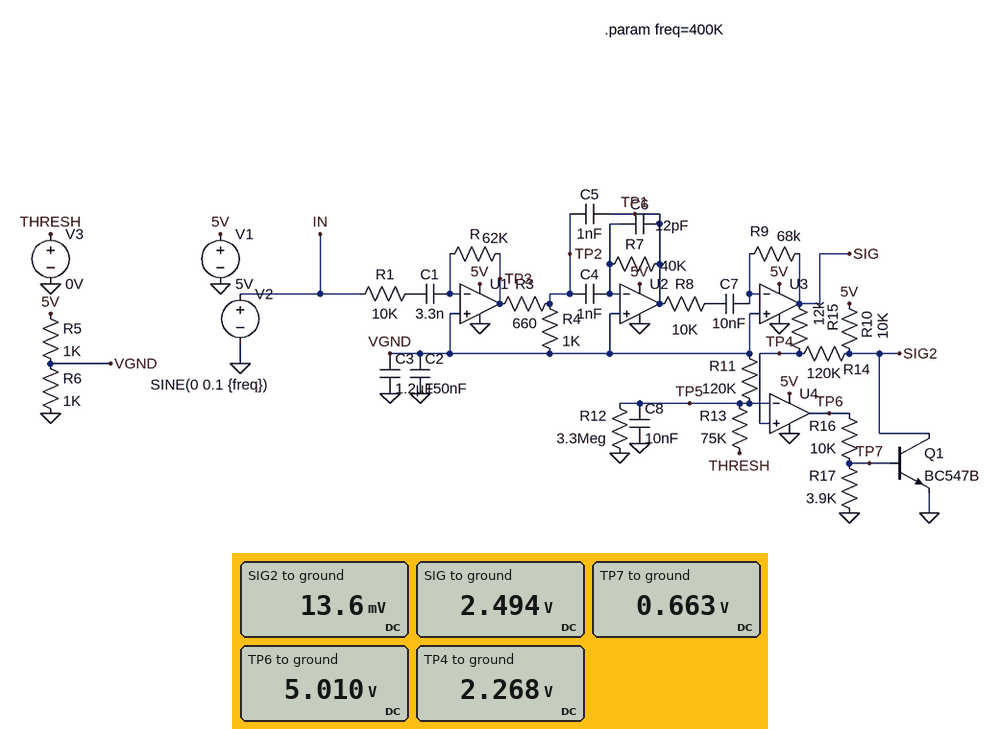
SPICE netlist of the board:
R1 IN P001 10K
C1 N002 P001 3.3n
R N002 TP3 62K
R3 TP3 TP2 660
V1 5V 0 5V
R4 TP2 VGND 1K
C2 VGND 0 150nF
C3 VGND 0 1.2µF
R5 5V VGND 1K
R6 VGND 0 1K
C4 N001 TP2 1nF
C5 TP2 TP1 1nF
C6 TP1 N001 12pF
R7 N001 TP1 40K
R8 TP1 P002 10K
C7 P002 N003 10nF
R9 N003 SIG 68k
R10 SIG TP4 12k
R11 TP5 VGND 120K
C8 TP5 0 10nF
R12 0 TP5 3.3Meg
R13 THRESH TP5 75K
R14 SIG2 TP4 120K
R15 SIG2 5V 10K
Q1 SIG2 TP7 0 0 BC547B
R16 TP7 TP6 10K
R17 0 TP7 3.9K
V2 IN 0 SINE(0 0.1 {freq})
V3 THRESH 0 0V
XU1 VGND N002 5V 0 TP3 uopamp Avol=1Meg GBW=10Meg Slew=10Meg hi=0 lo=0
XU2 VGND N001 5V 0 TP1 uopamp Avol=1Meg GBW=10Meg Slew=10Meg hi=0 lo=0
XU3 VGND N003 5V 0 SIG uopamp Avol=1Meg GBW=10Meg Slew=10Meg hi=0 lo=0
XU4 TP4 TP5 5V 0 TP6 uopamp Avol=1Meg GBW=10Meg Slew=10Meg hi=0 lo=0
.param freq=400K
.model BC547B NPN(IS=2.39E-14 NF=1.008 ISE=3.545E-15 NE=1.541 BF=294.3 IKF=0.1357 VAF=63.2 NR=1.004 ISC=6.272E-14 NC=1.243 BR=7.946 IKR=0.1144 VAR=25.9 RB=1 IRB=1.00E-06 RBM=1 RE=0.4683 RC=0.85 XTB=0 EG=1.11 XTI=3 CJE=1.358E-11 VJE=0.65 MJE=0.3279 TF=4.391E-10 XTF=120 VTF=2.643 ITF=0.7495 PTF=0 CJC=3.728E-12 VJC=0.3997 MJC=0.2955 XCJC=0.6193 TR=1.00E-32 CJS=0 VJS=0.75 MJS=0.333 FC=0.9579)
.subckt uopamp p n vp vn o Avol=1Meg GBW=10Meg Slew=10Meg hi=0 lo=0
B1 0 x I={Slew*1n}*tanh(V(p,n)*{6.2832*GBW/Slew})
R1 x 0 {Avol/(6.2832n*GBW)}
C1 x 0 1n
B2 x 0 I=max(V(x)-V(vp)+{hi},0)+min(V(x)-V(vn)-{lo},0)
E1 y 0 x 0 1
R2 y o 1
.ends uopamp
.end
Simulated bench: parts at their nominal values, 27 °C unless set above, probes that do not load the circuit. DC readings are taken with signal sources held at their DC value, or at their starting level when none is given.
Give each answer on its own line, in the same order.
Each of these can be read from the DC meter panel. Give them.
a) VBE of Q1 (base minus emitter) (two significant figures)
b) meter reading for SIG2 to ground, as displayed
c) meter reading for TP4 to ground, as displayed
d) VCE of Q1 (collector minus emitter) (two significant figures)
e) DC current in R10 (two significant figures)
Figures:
660 mV
13.6 mV
2.268 V
14 mV
19 µA
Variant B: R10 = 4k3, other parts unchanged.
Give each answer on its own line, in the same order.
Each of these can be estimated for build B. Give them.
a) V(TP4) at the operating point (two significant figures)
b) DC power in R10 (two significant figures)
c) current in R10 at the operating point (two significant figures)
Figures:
2.4 V
1.7 µW
20 µA
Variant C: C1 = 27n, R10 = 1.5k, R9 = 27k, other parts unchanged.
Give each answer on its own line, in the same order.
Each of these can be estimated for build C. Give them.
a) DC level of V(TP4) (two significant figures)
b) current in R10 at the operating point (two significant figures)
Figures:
2.5 V
20 µA
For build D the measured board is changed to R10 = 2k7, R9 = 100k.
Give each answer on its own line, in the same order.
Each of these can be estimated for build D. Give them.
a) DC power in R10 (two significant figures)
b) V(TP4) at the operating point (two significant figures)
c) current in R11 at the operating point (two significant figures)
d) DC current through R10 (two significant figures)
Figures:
1.1 µW
2.4 V
13 µA
20 µA
